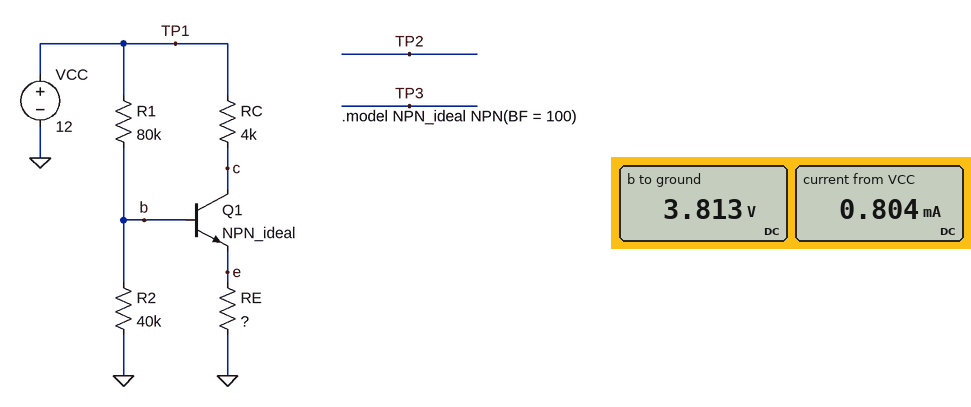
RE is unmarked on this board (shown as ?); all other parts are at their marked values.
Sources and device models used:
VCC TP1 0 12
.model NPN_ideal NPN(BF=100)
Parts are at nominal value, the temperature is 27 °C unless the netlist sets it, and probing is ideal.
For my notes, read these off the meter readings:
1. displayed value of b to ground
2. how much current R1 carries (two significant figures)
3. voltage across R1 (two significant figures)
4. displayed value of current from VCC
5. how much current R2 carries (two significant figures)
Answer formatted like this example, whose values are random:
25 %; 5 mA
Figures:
3.813 V; 100 µA; 8.2 V; 0.804 mA; 95 µA
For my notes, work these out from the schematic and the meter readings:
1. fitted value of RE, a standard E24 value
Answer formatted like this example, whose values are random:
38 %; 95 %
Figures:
4.3 kΩ
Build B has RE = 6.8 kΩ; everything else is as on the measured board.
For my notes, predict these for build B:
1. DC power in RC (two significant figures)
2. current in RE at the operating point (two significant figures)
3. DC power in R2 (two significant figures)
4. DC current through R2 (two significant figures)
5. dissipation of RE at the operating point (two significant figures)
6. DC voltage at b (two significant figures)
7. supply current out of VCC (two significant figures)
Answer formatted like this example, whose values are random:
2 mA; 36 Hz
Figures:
830 µW; 460 µA; 380 µW; 97 µA; 1.4 mW; 3.9 V; 560 µA
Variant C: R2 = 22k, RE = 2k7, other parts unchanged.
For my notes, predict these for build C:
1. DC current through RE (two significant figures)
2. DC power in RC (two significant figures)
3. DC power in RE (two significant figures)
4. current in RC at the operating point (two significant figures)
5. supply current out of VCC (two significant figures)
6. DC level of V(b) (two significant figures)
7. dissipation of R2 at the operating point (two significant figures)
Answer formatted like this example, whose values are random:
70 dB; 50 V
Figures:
640 µA; 1.6 mW; 1.1 mW; 630 µA; 750 µA; 2.5 V; 280 µW
